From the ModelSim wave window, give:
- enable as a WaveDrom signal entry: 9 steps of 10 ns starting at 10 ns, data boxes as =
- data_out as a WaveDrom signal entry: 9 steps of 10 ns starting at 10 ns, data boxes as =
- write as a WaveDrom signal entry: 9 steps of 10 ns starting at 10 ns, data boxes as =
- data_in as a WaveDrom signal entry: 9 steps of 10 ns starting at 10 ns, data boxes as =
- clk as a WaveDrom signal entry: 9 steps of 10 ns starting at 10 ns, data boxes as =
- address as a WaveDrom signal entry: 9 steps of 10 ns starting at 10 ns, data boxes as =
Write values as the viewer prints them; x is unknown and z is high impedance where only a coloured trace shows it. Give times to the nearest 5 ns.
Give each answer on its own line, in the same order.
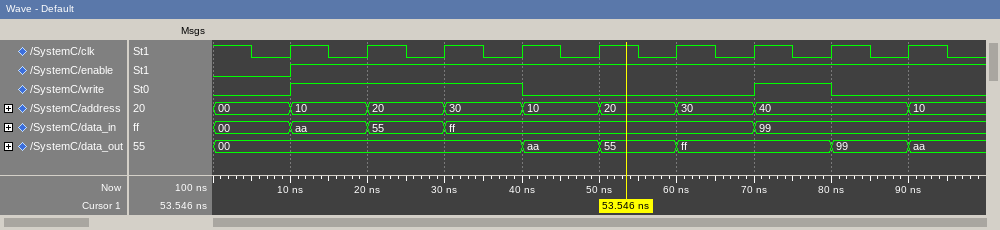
{name: 'enable', wave: '1........'}
{name: 'data_out', wave: '=..===.==', data: '00 aa 55 ff 99 aa'}
{name: 'write', wave: '1..0..10.'}
{name: 'data_in', wave: '===...=..', data: 'aa 55 ff 99'}
{name: 'clk', wave: 'p........'}
{name: 'address', wave: '=======.=', data: '10 20 30 10 20 30 40 10'}
